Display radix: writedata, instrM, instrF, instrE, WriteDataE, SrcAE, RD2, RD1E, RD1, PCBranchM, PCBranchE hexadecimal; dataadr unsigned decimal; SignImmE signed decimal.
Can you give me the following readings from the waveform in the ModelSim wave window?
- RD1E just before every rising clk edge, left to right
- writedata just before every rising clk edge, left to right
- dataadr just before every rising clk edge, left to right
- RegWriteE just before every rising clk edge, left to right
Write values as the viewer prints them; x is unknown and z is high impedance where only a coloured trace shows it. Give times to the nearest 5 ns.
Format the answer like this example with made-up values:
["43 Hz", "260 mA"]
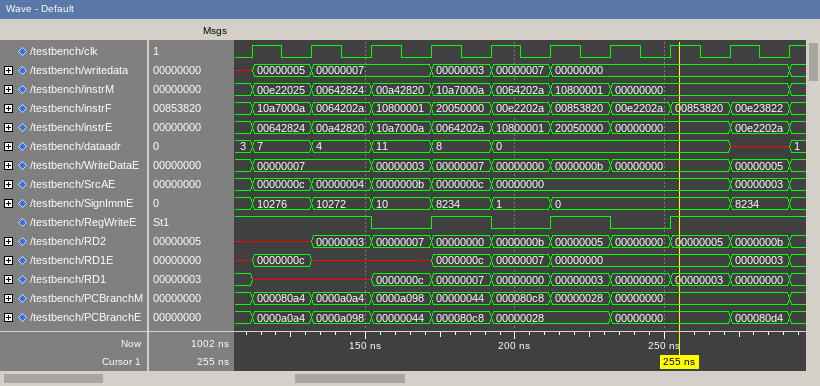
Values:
["x, 0000000c, x, x, 0000000c, 00000007, 00000000, 00000000, 00000000, 00000003", "x, 00000005, 00000007, 00000007, 00000003, 00000007, 00000000, 00000000, 00000000, 00000000", "3, 7, 4, 11, 8, 0, 0, 0, 0, x", "1 1 1 0 1 0 1 0 1 1"]
